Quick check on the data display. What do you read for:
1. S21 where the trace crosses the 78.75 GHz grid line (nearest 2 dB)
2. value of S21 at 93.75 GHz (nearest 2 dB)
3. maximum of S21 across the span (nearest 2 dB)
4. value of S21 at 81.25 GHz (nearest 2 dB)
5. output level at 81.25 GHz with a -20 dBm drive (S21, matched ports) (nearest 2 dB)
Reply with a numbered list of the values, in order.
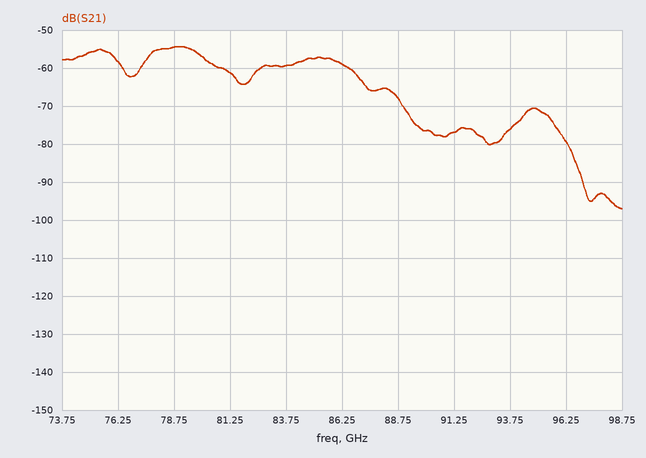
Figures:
1. -54 dB
2. -76 dB
3. -54 dB
4. -62 dB
5. -82 dBm
